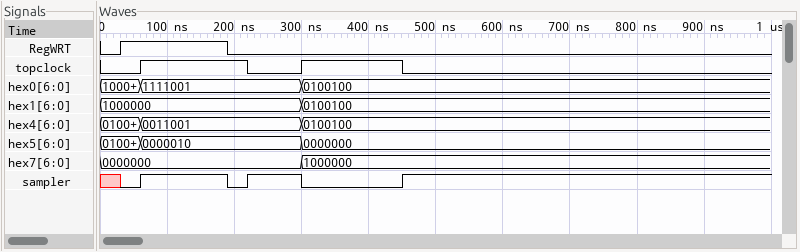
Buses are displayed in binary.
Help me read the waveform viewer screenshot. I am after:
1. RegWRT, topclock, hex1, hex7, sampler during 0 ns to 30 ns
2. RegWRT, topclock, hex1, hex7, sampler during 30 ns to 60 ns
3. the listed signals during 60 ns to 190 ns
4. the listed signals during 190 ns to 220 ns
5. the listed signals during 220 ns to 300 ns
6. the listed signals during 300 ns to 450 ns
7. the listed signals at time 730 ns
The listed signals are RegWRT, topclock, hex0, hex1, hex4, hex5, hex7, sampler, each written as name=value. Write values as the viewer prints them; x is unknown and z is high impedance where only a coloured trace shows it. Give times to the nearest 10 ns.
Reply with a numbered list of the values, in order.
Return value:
1. RegWRT=0, topclock=0, hex1=1000000, hex7=0000000, sampler=x
2. RegWRT=1, topclock=0, hex1=1000000, hex7=0000000, sampler=0
3. RegWRT=1, topclock=1, hex0=1111001, hex1=1000000, hex4=0011001, hex5=0000010, hex7=0000000, sampler=1
4. RegWRT=0, topclock=1, hex0=1111001, hex1=1000000, hex4=0011001, hex5=0000010, hex7=0000000, sampler=0
5. RegWRT=0, topclock=0, hex0=1111001, hex1=1000000, hex4=0011001, hex5=0000010, hex7=0000000, sampler=1
6. RegWRT=0, topclock=1, hex0=0100100, hex1=0100100, hex4=0100100, hex5=0000000, hex7=1000000, sampler=0
7. RegWRT=0, topclock=0, hex0=0100100, hex1=0100100, hex4=0100100, hex5=0000000, hex7=1000000, sampler=1
